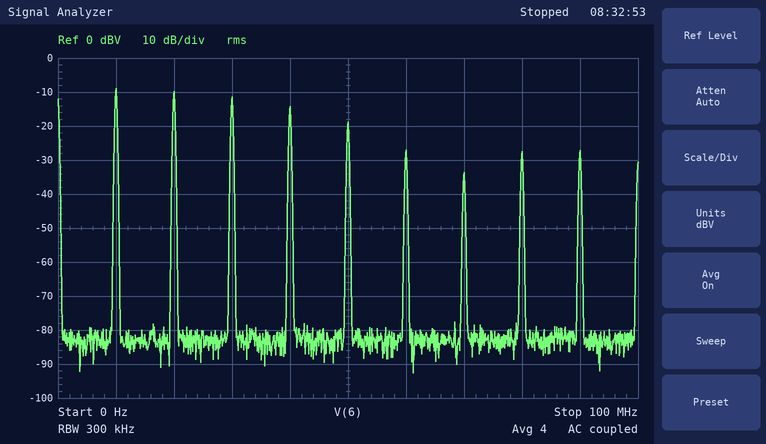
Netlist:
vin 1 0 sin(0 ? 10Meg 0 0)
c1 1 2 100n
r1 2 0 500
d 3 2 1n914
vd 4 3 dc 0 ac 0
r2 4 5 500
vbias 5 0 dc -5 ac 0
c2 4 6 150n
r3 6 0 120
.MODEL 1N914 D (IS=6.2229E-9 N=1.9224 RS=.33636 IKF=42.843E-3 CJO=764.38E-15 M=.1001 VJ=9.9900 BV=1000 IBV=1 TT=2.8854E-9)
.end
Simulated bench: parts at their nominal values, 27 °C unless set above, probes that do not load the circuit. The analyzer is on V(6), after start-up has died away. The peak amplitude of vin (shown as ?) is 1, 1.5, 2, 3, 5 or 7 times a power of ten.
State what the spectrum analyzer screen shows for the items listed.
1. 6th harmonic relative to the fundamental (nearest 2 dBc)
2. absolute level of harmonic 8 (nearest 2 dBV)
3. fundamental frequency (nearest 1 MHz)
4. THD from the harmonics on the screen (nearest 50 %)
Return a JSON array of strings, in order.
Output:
["-18 dBc", "-28 dBV", "10 MHz", "150 %"]
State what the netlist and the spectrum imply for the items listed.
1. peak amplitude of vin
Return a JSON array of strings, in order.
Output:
["10 V"]
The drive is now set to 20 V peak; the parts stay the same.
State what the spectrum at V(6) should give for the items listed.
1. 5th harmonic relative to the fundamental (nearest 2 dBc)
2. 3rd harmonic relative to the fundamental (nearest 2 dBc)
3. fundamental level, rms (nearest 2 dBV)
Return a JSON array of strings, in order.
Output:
["-18 dBc", "-4 dBc", "2 dBV"]
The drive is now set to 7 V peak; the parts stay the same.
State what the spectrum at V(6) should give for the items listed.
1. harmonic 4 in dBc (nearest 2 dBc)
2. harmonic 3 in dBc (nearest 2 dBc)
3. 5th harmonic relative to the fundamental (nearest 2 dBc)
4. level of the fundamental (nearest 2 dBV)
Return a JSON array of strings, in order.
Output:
["-2 dBc", "-2 dBc", "-4 dBc", "-20 dBV"]
